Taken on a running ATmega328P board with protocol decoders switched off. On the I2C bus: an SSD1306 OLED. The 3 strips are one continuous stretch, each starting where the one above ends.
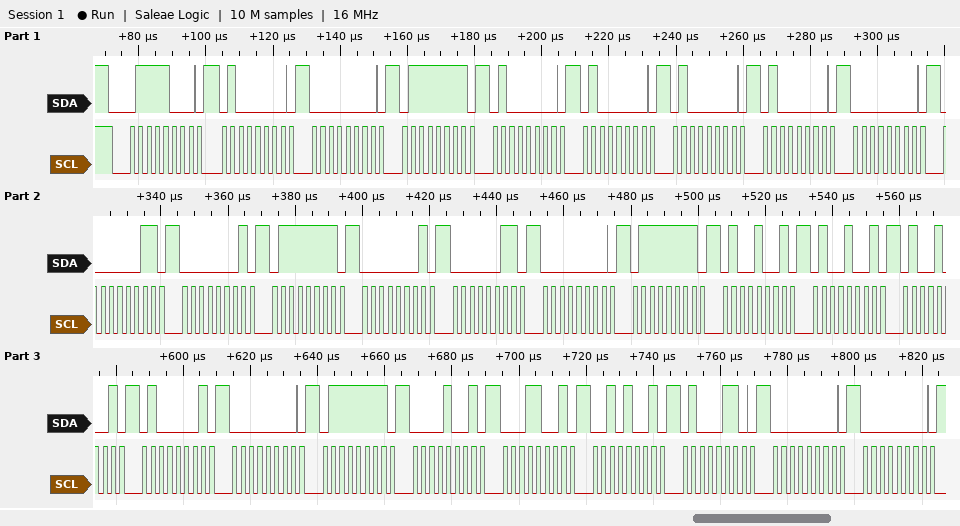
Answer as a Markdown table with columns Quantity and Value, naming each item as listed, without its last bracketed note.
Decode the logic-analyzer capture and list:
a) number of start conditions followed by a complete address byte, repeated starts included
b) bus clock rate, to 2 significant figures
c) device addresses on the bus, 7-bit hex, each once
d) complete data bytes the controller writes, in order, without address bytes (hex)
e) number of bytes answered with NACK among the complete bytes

| Quantity | Value |
|---|---|
| number of start conditions followed by a complete address byte, repeated starts included | 1 |
| bus clock rate, to 2 significant figures | 400 kHz |
| device addresses on the bus, 7-bit hex, each once | 0x3C |
| complete data bytes the controller writes, in order, without address bytes | 40 00 7F 40 40 40 40 00 03 01 7F 01 03 00 7F 49 49 49 41 00 7F 09 19 29 46 00 00 |
| number of bytes answered with NACK among the complete bytes | 0 |
